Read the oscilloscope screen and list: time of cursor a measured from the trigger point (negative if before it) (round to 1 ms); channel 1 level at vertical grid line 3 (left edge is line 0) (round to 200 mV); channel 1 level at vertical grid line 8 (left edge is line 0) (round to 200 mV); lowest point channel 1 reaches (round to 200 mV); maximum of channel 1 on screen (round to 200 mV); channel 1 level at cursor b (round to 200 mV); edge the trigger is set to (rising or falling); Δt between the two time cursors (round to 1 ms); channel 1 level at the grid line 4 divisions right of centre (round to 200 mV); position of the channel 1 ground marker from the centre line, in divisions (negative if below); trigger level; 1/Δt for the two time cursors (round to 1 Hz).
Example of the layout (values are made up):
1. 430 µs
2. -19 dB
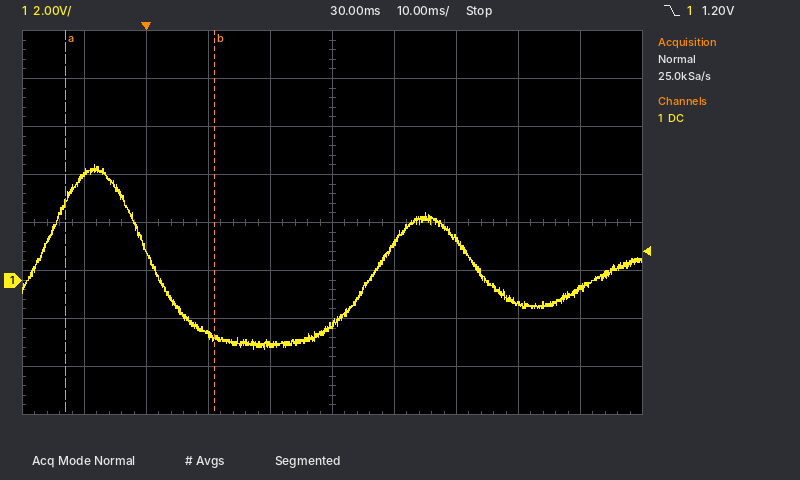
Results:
1. -13 ms
2. -2.2 V
3. -1.0 V
4. -2.8 V
5. 4.8 V
6. -2.4 V
7. falling
8. 24 ms
9. -400 mV
10. -1.2 div
11. 1.20 V
12. 42 Hz
